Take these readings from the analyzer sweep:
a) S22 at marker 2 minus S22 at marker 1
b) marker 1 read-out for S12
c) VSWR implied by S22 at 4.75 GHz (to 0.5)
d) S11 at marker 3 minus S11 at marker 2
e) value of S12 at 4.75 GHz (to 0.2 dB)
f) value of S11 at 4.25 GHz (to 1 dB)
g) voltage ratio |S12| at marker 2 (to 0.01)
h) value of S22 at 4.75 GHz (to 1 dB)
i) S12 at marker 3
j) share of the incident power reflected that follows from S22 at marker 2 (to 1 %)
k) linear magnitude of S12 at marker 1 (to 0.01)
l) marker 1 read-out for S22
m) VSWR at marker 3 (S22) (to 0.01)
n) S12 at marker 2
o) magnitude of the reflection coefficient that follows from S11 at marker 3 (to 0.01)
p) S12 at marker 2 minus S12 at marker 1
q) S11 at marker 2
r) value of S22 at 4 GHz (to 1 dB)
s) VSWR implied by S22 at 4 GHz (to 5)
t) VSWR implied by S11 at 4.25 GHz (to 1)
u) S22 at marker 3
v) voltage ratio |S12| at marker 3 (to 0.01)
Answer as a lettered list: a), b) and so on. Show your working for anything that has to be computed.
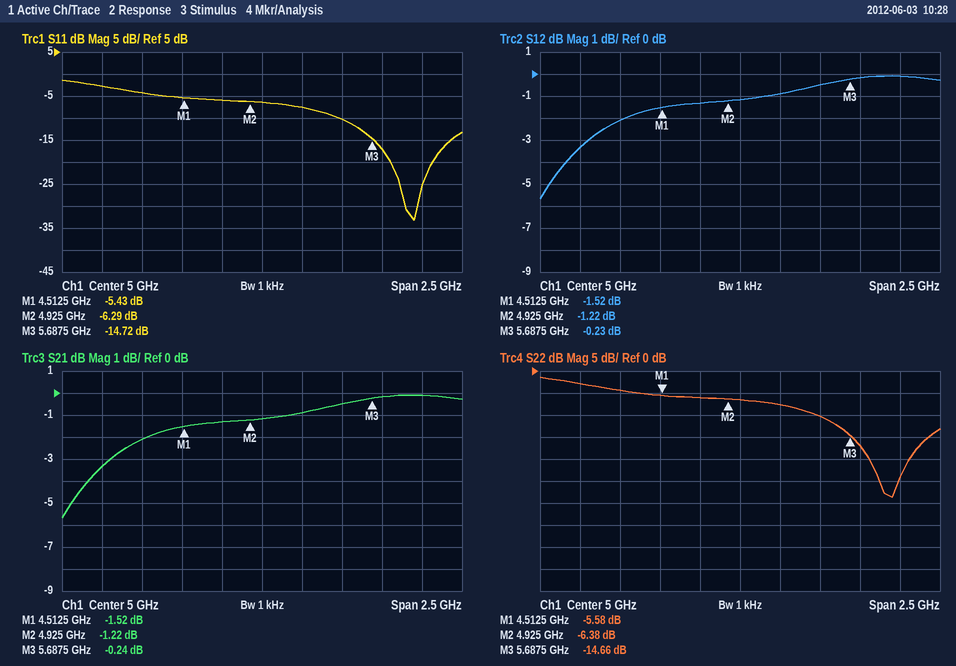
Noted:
a) -6.38 − (-5.58) = -0.80 dB
b) -1.52 dB
c) |Γ| = 10^(-6/20) = 0.5012; VSWR = (1 + 0.5012)/(1 − 0.5012) ≈ 3.0
d) -14.72 − (-6.29) = -8.43 dB
e) -1.4 dB
f) -4 dB
g) 10^(-1.22/20) ≈ 0.87
h) -6 dB
i) -0.23 dB
j) 10^(-6.38/10) ≈ 23 %
k) 10^(-1.52/20) ≈ 0.84
l) -5.58 dB
m) (1 + 0.1849)/(1 − 0.1849) ≈ 1.45
n) -1.22 dB
o) 10^(-14.72/20) ≈ 0.18
p) -1.22 − (-1.52) = 0.30 dB
q) -6.29 dB
r) -3 dB
s) |Γ| = 10^(-3/20) = 0.7079; VSWR = (1 + 0.7079)/(1 − 0.7079) ≈ 5.85, so 5 to the nearest 5
t) |Γ| = 10^(-4/20) = 0.6310; VSWR = (1 + 0.6310)/(1 − 0.6310) ≈ 4
u) -14.66 dB
v) 10^(-0.23/20) ≈ 0.97
